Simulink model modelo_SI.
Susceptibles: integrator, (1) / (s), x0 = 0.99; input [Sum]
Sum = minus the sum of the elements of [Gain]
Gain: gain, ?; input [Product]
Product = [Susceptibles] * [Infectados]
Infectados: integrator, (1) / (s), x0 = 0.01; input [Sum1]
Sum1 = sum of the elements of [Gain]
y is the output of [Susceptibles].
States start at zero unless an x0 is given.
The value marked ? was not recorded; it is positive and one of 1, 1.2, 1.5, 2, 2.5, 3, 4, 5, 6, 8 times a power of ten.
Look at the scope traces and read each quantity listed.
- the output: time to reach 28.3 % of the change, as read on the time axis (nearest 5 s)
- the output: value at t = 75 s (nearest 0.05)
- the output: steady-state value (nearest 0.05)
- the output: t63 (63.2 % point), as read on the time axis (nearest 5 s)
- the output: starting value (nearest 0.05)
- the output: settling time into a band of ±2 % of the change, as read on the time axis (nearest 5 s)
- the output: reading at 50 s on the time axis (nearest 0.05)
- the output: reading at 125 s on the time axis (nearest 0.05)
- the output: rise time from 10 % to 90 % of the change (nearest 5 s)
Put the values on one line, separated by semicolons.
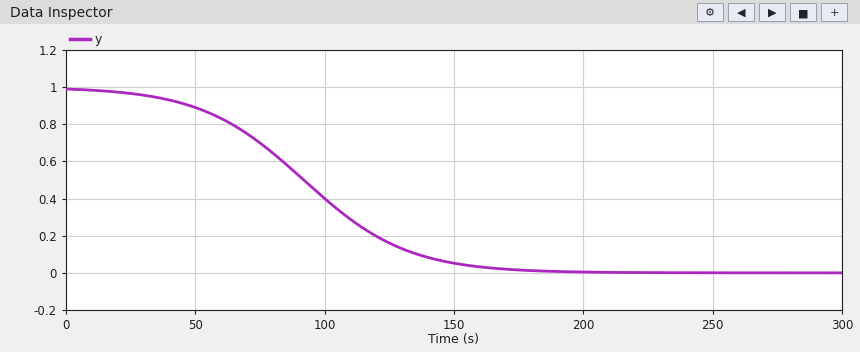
75 s; 0.70; 0.00; 105 s; 1.00; 170 s; 0.90; 0.15; 85 s
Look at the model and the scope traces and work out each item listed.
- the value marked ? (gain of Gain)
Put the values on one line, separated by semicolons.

0.05
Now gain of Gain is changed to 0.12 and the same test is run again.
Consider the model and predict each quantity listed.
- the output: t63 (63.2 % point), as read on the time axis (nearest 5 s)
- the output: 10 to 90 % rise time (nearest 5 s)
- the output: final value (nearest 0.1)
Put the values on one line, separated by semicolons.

45 s; 35 s; 0.0
